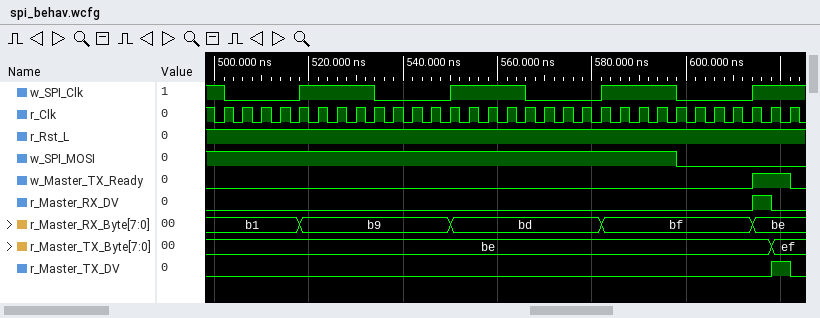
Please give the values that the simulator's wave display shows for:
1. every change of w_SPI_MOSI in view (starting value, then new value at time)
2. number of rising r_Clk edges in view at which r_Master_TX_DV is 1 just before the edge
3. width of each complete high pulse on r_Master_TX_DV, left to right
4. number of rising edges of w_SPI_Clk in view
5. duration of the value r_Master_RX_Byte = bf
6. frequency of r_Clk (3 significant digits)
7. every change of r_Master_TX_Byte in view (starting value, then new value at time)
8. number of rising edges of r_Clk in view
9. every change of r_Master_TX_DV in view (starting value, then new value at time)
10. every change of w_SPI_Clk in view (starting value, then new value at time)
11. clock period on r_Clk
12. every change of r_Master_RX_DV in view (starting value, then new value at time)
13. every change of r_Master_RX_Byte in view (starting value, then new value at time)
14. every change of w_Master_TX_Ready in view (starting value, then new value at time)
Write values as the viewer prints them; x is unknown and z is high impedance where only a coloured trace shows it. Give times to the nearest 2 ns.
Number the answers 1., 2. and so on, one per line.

1. 1, 0 at 598 ns
2. 1
3. 4 ns
4. 4
5. 32 ns
6. 250 MHz
7. be, ef at 618 ns
8. 31
9. 0, 1 at 618 ns, 0 at 622 ns
10. 1, 0 at 502 ns, 1 at 518 ns, 0 at 534 ns, 1 at 550 ns, 0 at 566 ns, 1 at 582 ns, 0 at 598 ns, 1 at 614 ns
11. 4 ns
12. 0, 1 at 614 ns, 0 at 618 ns
13. b1, b9 at 518 ns, bd at 550 ns, bf at 582 ns, be at 614 ns
14. 0, 1 at 614 ns, 0 at 622 ns
